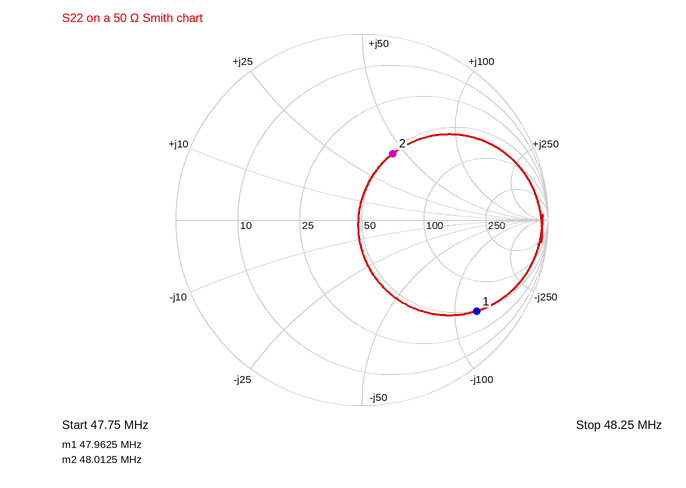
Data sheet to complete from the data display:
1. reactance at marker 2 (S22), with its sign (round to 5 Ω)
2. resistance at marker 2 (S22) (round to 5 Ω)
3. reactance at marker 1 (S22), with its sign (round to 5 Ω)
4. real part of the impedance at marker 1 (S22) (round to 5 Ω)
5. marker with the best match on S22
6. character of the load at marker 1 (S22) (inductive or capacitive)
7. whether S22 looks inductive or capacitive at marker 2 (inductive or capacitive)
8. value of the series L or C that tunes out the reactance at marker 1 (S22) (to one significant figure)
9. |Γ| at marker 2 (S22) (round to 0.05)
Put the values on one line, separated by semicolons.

+45 Ω; 50 Ω; -125 Ω; 50 Ω; marker 2; capacitive; inductive; 400 nH; 0.40
